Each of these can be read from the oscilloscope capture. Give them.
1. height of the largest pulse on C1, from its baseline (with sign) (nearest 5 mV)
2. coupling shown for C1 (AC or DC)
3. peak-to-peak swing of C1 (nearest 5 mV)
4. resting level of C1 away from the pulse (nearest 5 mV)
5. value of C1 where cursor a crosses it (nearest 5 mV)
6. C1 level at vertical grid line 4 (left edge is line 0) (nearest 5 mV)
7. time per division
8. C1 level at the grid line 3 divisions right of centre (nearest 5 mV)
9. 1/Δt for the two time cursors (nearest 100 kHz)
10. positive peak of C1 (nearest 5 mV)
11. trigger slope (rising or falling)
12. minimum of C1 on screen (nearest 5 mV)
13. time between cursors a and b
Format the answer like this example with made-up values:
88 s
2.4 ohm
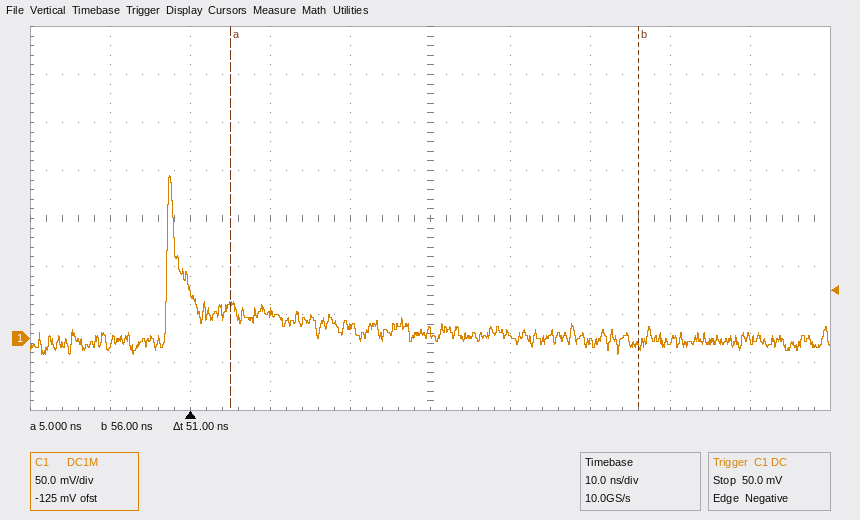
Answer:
+170 mV
DC
185 mV
0 mV
35 mV
15 mV
10 ns
0 mV
19.6 MHz
170 mV
falling
-15 mV
51 ns
